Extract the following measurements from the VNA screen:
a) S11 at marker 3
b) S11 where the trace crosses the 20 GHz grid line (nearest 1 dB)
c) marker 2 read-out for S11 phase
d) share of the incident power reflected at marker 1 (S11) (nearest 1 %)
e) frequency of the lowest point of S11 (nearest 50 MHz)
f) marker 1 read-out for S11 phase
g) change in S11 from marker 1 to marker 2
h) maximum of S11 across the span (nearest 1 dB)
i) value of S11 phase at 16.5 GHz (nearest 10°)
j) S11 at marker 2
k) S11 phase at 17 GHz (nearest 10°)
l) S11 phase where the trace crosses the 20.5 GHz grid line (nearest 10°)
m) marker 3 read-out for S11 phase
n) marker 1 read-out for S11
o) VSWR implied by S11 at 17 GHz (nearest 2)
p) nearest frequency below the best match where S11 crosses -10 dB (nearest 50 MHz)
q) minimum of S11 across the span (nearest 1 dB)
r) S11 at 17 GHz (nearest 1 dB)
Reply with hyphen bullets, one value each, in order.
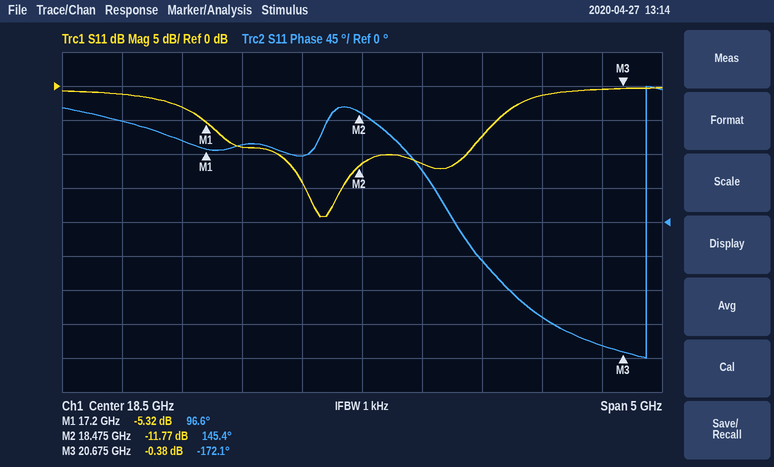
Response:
- -0.38 dB
- -1 dB
- 145.4°
- 29 %
- 18.15 GHz
- 96.6°
- -6.45 dB
- 0 dB
- 130°
- -11.77 dB
- 110°
- -160°
- -172.1°
- -5.32 dB
- 6
- 17.80 GHz
- -19 dB
- -3 dB
